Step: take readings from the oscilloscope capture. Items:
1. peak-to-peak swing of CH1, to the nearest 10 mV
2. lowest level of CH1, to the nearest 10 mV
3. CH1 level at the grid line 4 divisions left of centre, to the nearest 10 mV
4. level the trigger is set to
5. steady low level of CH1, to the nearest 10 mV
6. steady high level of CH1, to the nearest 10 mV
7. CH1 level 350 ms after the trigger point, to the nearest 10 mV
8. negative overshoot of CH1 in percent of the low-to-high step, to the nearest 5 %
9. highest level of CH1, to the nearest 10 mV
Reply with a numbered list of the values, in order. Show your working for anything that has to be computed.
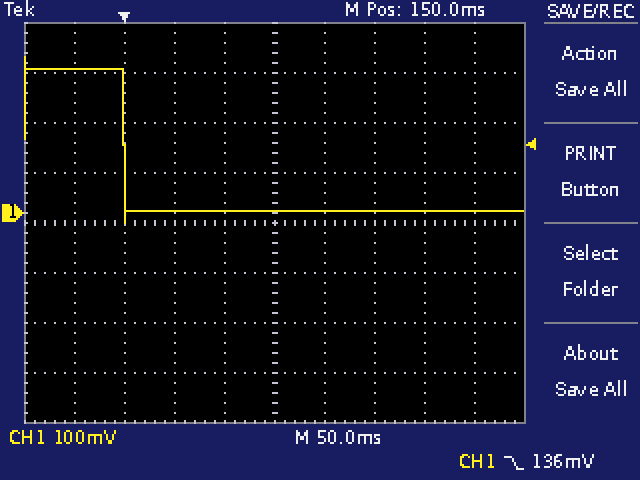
1. 310 mV − (-20 mV) = 330 mV
2. -20 mV
3. 290 mV
4. 136 mV
5. 0 mV
6. 290 mV
7. 0 mV
8. 10 %
9. 310 mV
